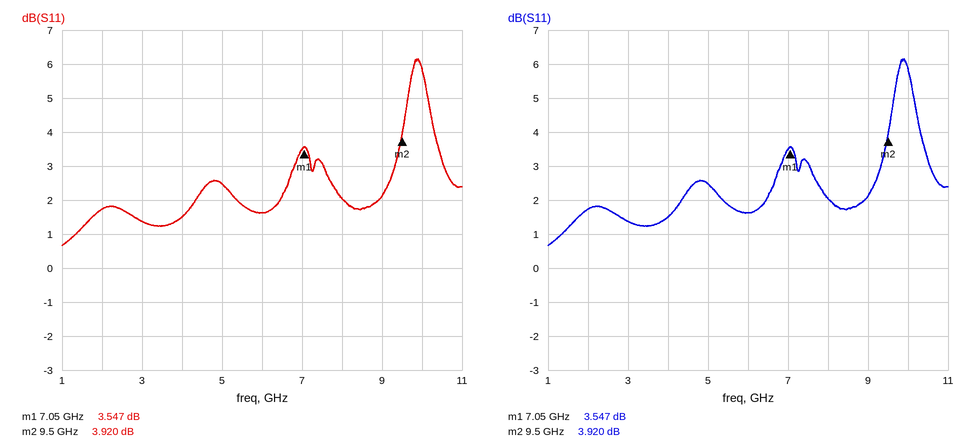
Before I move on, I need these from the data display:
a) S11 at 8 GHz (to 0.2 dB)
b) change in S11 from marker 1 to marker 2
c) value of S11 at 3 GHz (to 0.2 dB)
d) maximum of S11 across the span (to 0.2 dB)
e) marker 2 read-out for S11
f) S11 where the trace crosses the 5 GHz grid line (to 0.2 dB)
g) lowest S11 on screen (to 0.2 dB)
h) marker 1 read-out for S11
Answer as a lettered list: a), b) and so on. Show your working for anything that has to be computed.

a) 2.0 dB
b) 3.92 − (3.547) = 0.373 dB
c) 1.4 dB
d) 6.2 dB
e) 3.920 dB
f) 2.4 dB
g) 0.6 dB
h) 3.547 dB
